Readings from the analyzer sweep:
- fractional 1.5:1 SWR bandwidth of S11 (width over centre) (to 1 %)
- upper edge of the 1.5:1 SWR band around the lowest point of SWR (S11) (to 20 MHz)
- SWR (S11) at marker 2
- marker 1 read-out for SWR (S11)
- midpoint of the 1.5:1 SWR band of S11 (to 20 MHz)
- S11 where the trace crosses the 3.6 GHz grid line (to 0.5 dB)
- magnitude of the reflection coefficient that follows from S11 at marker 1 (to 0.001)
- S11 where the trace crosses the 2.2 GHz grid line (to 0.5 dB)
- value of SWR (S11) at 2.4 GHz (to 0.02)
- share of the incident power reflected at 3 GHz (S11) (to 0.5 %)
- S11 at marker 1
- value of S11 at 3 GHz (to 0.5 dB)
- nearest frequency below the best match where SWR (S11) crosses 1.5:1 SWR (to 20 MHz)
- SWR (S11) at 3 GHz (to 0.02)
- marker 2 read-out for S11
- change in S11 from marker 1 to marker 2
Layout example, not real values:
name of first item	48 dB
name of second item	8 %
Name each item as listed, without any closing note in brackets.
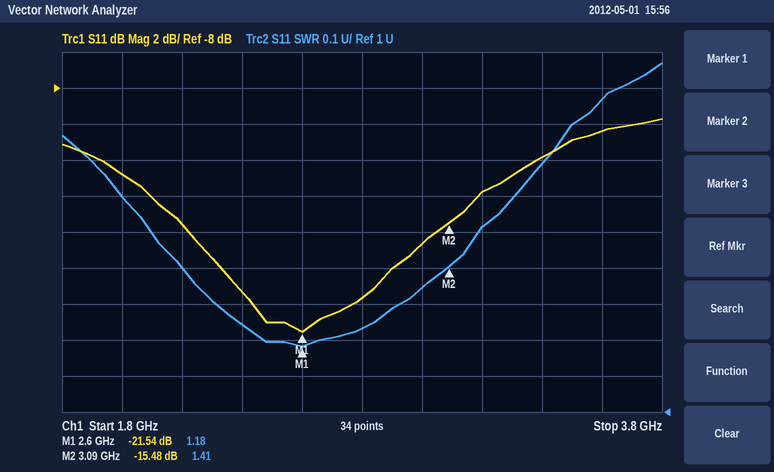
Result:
fractional 1.5:1 SWR bandwidth of S11 (width over centre)	41 %
upper edge of the 1.5:1 SWR band around the lowest point of SWR (S11)	3.18 GHz
SWR (S11) at marker 2	1.41
marker 1 read-out for SWR	1.18
midpoint of the 1.5:1 SWR band of S11	2.64 GHz
S11 where the trace crosses the 3.6 GHz grid line	-10.5 dB
magnitude of the reflection coefficient that follows from S11 at marker 1	0.084
S11 where the trace crosses the 2.2 GHz grid line	-15.5 dB
value of SWR (S11) at 2.4 GHz	1.24
share of the incident power reflected at 3 GHz (S11)	2.0 %
S11 at marker 1	-21.54 dB
value of S11 at 3 GHz	-16.5 dB
nearest frequency below the best match where SWR (S11) crosses 1.5:1 SWR	2.10 GHz
SWR (S11) at 3 GHz	1.34
marker 2 read-out for S11	-15.48 dB
change in S11 from marker 1 to marker 2	6.06 dB
